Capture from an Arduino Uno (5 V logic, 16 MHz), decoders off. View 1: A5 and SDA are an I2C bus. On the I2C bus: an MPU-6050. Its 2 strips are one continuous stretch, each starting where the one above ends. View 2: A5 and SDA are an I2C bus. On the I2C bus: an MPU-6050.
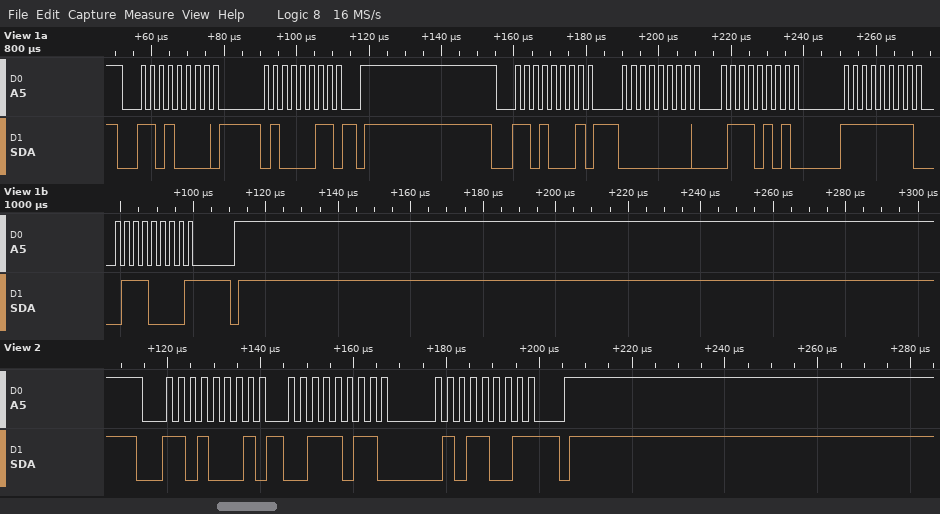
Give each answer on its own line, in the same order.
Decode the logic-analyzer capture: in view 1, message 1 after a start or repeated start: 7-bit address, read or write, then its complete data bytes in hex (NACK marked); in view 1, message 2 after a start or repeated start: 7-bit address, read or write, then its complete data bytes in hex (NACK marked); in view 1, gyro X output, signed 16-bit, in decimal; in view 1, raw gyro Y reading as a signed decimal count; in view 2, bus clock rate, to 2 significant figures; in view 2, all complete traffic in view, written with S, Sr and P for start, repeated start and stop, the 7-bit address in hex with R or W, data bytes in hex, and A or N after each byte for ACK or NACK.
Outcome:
0x68 write: 43
0x68 read: 00 75 FF 70 NACK
117
-144
400 kHz
S 68R A 3B A 59 N P
